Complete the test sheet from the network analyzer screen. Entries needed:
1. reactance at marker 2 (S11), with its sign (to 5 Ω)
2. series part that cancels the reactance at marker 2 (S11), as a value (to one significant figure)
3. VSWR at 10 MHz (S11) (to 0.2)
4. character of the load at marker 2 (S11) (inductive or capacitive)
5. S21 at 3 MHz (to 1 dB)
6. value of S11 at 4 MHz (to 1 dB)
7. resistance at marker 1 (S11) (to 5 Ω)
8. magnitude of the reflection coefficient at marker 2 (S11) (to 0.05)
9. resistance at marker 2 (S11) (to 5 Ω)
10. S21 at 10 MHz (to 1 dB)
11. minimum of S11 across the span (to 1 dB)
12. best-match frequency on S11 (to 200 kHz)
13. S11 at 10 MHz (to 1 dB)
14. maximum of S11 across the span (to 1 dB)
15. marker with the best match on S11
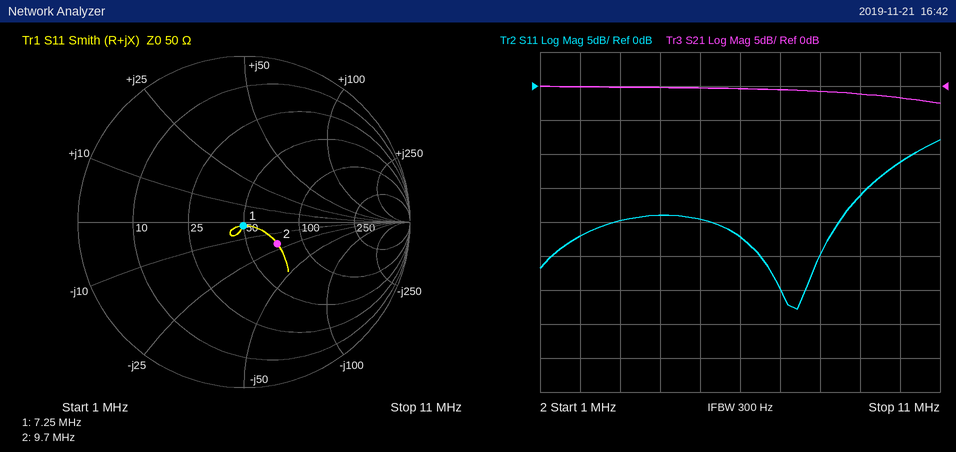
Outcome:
-20 Ω
300 nH
1.8
capacitive
0 dB
-19 dB
50 Ω
0.25
70 Ω
-2 dB
-33 dB
7.4 MHz
-11 dB
-8 dB
marker 1
